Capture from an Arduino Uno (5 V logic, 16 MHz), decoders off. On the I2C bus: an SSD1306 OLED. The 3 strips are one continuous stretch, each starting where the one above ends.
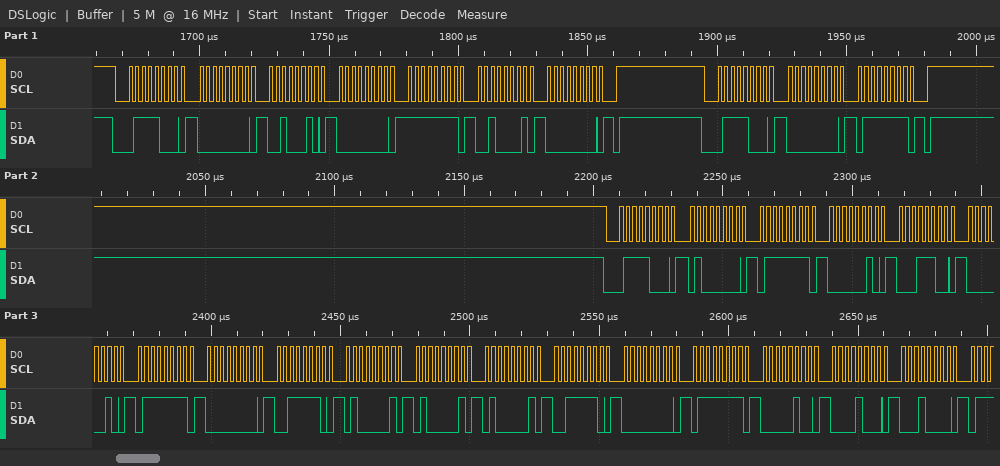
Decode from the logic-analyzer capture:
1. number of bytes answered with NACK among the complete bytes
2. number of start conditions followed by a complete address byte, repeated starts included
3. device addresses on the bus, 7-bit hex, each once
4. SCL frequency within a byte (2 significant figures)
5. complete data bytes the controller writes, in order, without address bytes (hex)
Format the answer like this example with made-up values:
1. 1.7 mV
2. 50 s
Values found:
1. 0
2. 3
3. 0x3C
4. 400 kHz
5. 00 22 00 FF 21 00 00 7F 40 7F 02 1C 02 7F 00 3E 41 41 41 3E 00 7F 04 08 10
